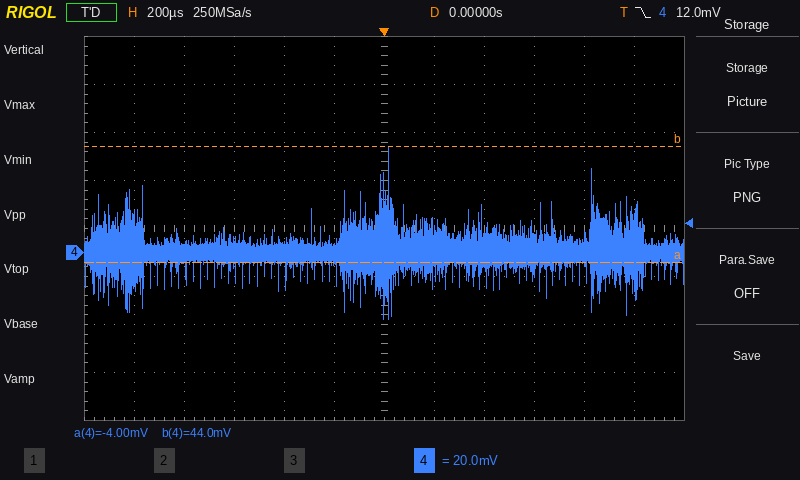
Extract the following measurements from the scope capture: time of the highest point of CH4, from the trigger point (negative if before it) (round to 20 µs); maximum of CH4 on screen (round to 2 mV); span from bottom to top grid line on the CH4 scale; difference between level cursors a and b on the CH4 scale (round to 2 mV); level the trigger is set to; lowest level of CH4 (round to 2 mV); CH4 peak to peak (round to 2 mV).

+20 µs
44 mV
160 mV
48 mV
12.0 mV
-28 mV
72 mV
